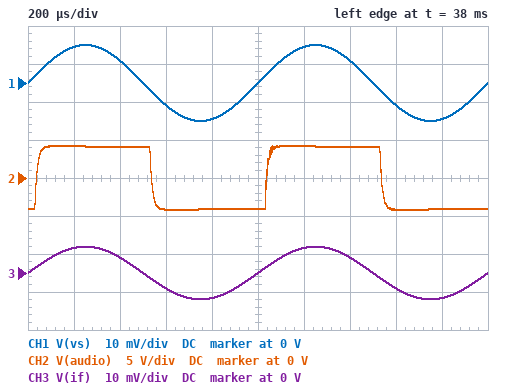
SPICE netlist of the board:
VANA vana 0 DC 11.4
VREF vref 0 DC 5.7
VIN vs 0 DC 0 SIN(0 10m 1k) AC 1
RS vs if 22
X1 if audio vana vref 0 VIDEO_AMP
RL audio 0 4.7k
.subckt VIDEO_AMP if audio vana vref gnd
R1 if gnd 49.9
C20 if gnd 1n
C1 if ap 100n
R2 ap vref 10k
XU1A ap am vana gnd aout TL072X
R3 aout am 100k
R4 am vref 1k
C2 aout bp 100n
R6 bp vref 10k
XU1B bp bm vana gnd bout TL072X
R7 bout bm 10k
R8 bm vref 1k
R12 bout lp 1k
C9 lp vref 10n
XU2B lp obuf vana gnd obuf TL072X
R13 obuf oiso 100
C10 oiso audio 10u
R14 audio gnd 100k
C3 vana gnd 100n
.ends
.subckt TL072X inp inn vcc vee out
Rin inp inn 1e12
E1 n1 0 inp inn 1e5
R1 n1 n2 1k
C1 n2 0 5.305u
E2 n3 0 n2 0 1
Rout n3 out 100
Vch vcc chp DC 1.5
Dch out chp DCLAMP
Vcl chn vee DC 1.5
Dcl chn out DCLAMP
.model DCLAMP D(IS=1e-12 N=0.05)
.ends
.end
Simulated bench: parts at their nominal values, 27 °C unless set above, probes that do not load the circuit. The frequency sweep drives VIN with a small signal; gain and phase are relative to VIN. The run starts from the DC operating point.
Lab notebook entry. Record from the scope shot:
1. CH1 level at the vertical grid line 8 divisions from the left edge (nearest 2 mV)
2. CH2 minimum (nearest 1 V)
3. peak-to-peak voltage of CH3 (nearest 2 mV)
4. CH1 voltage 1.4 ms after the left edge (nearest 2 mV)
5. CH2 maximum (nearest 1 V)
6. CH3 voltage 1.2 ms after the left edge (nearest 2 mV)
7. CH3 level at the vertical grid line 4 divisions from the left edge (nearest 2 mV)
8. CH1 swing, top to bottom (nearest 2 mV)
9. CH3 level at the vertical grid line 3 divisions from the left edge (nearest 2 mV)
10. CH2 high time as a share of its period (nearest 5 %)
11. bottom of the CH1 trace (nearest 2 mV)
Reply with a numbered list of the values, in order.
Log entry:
1. -6 mV
2. -4 V
3. 14 mV
4. 6 mV
5. 4 V
6. 6 mV
7. -6 mV
8. 20 mV
9. -4 mV
10. 50 %
11. -10 mV
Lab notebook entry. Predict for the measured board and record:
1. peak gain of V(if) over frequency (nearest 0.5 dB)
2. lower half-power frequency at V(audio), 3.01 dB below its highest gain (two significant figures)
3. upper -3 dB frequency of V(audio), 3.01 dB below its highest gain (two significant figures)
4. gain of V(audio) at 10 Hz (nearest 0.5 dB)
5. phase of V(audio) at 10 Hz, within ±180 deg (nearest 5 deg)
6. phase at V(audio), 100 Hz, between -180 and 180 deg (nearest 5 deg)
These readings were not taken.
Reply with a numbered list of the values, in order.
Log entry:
1. -3.0 dB
2. 240 Hz
3. 13 kHz
4. 9.0 dB
5. -170 deg
6. 115 deg
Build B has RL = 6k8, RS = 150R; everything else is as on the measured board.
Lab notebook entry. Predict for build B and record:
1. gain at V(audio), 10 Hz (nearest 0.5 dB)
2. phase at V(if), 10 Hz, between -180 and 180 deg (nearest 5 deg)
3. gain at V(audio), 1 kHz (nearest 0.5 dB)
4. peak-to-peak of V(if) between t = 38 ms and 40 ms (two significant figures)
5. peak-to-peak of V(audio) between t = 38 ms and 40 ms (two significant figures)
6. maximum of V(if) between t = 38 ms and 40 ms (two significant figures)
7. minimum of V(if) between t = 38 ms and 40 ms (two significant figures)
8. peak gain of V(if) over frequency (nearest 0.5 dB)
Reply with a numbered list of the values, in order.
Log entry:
1. 0.5 dB
2. 0 deg
3. 48.5 dB
4. 5.0 mV
5. 5.3 V
6. 2.5 mV
7. -2.5 mV
8. -12.0 dB
